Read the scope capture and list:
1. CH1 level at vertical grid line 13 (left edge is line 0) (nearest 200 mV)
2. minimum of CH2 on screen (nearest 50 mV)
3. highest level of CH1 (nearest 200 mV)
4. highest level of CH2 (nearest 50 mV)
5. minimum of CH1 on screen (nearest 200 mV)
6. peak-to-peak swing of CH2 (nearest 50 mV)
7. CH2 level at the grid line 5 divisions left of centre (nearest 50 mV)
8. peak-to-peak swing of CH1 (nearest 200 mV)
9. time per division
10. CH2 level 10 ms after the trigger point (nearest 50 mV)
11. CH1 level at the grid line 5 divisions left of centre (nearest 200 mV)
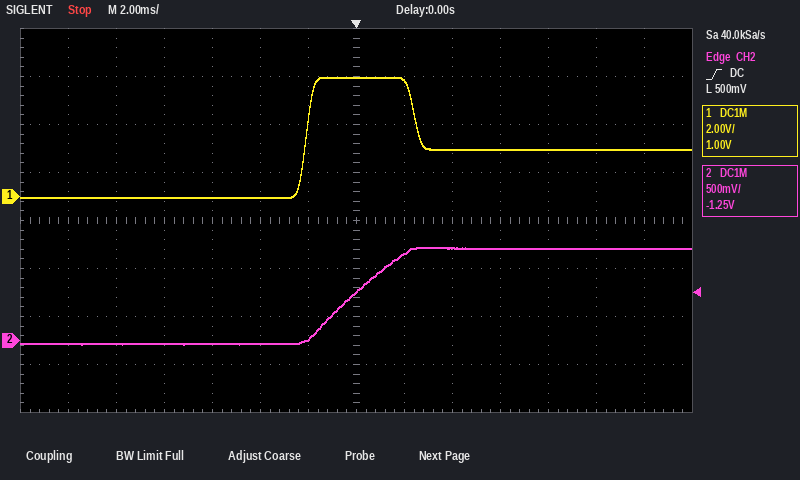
2.0 V
-50 mV
5.0 V
950 mV
0.0 V
1.00 V
-50 mV
5.0 V
2 ms
950 mV
0.0 V
